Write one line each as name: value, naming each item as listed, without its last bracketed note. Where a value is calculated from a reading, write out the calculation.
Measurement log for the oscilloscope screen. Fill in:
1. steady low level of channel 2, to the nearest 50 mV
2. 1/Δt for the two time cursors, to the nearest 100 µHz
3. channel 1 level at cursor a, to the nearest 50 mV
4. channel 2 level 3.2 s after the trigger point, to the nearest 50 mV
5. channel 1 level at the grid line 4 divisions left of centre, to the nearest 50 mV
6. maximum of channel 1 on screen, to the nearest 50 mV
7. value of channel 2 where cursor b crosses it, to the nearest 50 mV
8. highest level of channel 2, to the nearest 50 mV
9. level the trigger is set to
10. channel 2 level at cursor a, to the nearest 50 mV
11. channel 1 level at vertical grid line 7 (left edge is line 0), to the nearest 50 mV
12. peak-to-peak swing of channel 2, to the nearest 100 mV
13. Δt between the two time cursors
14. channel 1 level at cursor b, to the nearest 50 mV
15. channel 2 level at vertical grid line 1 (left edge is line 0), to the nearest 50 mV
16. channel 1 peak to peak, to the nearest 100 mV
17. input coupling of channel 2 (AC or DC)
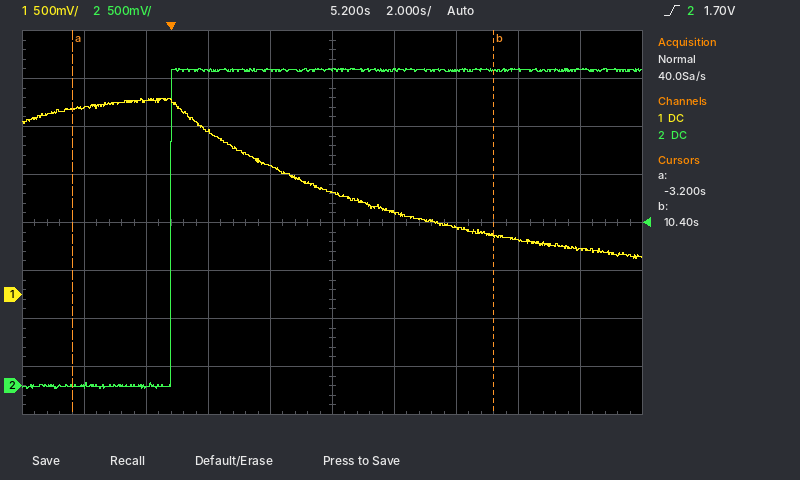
steady low level of channel 2, to the nearest 50 mV: 0 mV
1/Δt for the two time cursors, to the nearest 100 µHz: 1 / 13.6 s ≈ 73.5 mHz
channel 1 level at cursor a, to the nearest 50 mV: 1.95 V
channel 2 level 3.2 s after the trigger point, to the nearest 50 mV: 3.30 V
channel 1 level at the grid line 4 divisions left of centre, to the nearest 50 mV: 1.95 V
maximum of channel 1 on screen, to the nearest 50 mV: 2.05 V
value of channel 2 where cursor b crosses it, to the nearest 50 mV: 3.30 V
highest level of channel 2, to the nearest 50 mV: 3.30 V
level the trigger is set to: 1.70 V
channel 2 level at cursor a, to the nearest 50 mV: 0 mV
channel 1 level at vertical grid line 7 (left edge is line 0), to the nearest 50 mV: 700 mV
peak-to-peak swing of channel 2, to the nearest 100 mV: 3.30 V
Δt between the two time cursors: 10.4 s − (-3.2 s) = 13.6 s
channel 1 level at cursor b, to the nearest 50 mV: 600 mV
channel 2 level at vertical grid line 1 (left edge is line 0), to the nearest 50 mV: 0 mV
channel 1 peak to peak, to the nearest 100 mV: 1.70 V
input coupling of channel 2: DC
